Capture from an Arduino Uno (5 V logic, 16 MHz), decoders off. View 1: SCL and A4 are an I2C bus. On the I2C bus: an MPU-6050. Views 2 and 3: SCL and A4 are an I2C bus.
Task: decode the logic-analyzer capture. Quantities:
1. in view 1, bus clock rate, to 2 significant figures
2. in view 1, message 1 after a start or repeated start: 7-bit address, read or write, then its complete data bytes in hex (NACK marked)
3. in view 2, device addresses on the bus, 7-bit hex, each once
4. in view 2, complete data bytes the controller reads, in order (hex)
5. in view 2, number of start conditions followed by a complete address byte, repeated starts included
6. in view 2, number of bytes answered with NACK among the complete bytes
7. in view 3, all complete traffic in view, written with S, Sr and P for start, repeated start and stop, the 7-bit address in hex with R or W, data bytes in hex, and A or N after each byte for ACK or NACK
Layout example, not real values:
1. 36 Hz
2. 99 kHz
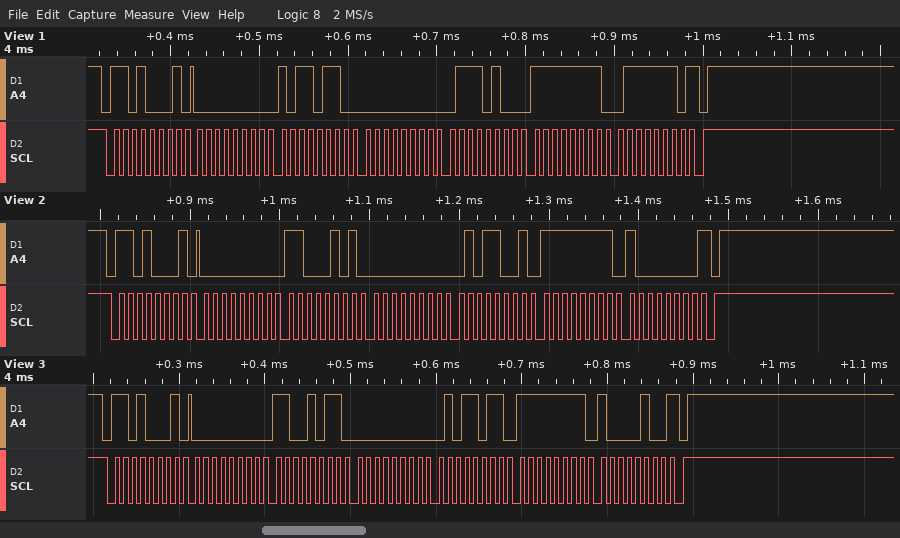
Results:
1. 100 kHz
2. 0x68 read: 00 B6 00 74 FF 7E NACK
3. 0x68
4. 00 C5 00 59 FF 80
5. 1
6. 1
7. S 68R A 00 A CB A 00 A 5B A FF A 84 N P
